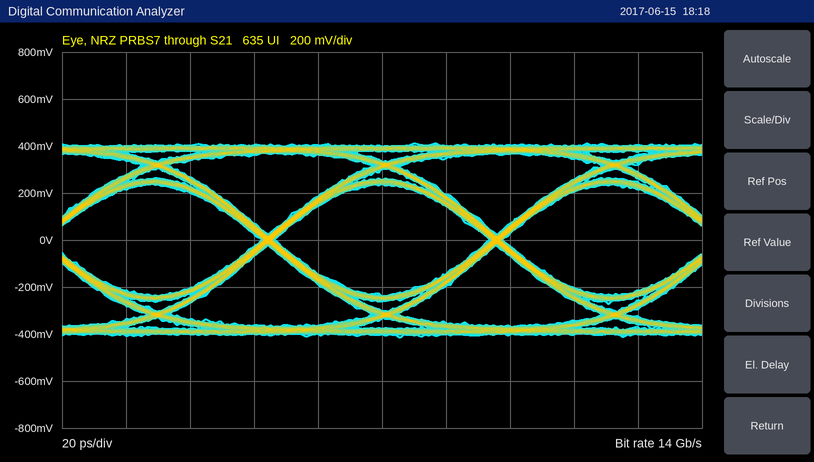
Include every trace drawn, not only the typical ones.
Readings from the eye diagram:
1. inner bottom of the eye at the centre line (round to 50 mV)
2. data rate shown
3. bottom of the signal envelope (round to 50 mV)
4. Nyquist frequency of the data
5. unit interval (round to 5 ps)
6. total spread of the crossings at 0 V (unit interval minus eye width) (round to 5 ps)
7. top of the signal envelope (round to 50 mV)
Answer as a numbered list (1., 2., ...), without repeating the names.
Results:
1. -250 mV
2. 14 Gb/s
3. -400 mV
4. 7 GHz
5. 70 ps
6. 5 ps
7. 400 mV
